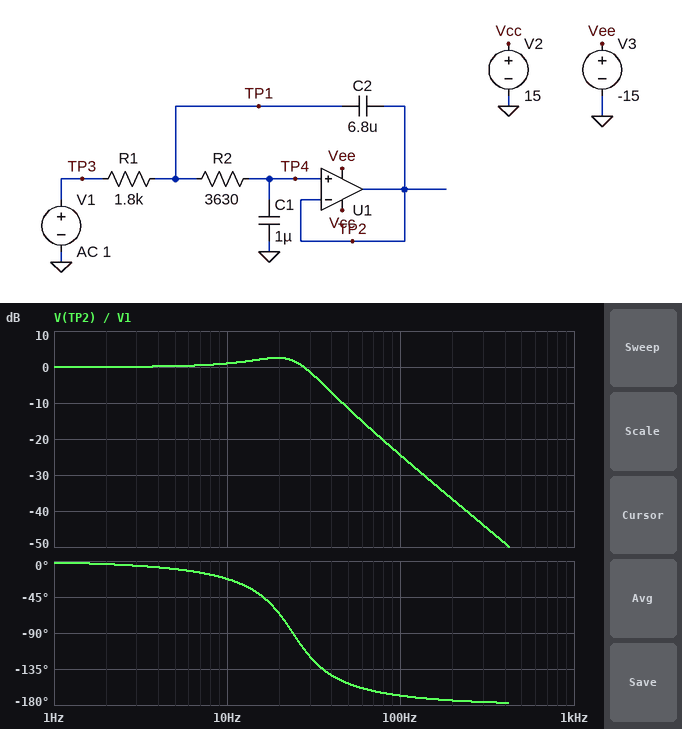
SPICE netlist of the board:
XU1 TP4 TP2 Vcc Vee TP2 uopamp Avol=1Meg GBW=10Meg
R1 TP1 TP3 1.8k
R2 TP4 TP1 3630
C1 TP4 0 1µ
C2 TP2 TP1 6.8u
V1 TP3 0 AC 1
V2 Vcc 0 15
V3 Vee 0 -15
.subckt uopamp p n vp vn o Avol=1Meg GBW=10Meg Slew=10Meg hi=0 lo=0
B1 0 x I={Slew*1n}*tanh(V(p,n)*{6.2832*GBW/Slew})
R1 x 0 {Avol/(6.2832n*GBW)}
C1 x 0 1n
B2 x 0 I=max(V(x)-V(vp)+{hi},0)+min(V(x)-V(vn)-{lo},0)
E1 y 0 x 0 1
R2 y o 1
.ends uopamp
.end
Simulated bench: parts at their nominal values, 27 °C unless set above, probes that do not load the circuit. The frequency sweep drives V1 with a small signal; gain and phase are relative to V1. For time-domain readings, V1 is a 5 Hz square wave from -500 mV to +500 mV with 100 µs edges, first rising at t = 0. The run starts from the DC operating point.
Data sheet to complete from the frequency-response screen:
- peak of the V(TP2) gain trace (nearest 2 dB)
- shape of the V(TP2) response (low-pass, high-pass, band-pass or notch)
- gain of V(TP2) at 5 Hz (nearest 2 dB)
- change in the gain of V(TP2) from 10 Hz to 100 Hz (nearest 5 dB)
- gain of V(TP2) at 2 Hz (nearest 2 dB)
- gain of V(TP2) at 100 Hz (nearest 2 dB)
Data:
2 dB
low-pass
0 dB
-25 dB
0 dB
-24 dB
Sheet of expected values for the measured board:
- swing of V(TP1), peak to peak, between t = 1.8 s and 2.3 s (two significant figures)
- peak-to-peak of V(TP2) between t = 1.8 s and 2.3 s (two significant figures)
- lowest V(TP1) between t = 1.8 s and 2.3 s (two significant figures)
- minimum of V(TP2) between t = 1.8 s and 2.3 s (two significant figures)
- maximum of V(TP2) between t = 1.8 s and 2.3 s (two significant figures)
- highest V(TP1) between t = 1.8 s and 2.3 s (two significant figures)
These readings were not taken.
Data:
1.6 V
1.5 V
-790 mV
-750 mV
750 mV
790 mV
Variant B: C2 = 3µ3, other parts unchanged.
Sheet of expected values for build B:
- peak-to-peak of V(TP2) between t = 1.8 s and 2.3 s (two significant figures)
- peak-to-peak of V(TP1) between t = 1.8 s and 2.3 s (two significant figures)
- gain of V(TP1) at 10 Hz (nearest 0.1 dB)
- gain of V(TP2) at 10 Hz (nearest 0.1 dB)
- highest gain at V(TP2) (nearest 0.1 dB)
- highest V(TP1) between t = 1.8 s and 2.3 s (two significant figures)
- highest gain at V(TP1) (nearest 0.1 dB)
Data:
1.2 V
1.3 V
0.4 dB
0.2 dB
0.5 dB
660 mV
1.5 dB
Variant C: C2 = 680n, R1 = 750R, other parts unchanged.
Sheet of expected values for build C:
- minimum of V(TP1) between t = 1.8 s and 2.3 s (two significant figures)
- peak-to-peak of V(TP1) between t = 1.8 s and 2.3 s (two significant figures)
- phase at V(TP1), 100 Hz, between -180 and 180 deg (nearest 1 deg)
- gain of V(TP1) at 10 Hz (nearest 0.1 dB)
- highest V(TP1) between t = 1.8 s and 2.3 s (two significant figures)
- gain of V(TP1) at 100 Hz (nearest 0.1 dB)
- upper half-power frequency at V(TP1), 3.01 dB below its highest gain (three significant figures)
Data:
-500 mV
1.0 V
-18 deg
0 dB
500 mV
-0.9 dB
287 Hz
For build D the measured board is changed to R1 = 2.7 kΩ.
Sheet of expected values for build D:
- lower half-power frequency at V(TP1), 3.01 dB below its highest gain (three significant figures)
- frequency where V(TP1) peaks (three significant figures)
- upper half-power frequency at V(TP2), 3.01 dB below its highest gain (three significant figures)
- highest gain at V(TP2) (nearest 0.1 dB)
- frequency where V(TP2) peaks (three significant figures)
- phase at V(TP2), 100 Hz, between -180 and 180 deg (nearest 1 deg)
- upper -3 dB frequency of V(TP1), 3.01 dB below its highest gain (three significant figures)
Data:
5.17 Hz
16.8 Hz
23.2 Hz
2.9 dB
16.3 Hz
-171 deg
23.9 Hz
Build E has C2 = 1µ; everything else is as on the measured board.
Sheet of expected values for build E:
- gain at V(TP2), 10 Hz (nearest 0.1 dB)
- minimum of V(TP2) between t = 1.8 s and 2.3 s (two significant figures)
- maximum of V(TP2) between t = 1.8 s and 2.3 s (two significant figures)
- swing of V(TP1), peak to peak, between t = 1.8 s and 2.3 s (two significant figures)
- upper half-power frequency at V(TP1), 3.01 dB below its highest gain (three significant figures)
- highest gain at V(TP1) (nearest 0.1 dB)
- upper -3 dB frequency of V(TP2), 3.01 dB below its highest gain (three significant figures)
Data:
-0.3 dB
-500 mV
500 mV
1.0 V
88.4 Hz
0 dB
36.8 Hz
